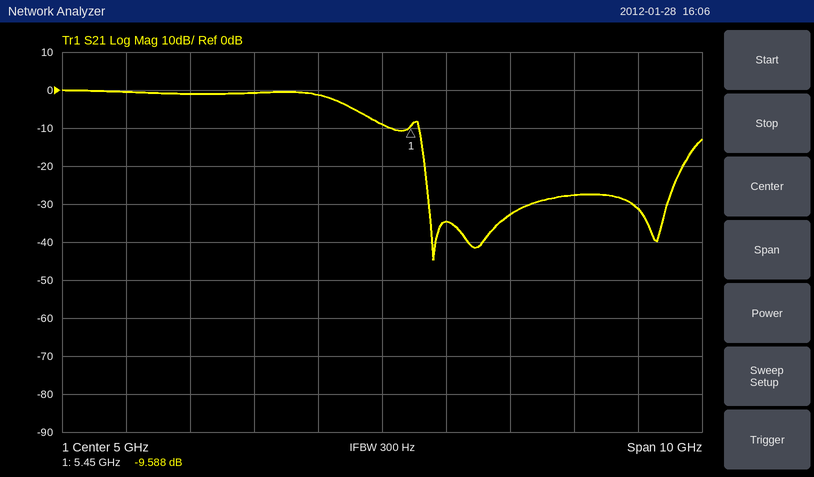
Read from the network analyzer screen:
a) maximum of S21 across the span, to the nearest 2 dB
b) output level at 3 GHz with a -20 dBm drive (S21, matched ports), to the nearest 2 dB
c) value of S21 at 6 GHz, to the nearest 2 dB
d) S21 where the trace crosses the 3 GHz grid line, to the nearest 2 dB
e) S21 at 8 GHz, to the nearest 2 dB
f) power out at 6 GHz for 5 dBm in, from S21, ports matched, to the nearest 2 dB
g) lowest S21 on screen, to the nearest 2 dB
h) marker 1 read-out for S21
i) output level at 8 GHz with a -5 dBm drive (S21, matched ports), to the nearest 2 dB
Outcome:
0 dB
-20 dBm
-34 dB
0 dB
-28 dB
-30 dBm
-44 dB
-9.588 dB
-32 dBm
